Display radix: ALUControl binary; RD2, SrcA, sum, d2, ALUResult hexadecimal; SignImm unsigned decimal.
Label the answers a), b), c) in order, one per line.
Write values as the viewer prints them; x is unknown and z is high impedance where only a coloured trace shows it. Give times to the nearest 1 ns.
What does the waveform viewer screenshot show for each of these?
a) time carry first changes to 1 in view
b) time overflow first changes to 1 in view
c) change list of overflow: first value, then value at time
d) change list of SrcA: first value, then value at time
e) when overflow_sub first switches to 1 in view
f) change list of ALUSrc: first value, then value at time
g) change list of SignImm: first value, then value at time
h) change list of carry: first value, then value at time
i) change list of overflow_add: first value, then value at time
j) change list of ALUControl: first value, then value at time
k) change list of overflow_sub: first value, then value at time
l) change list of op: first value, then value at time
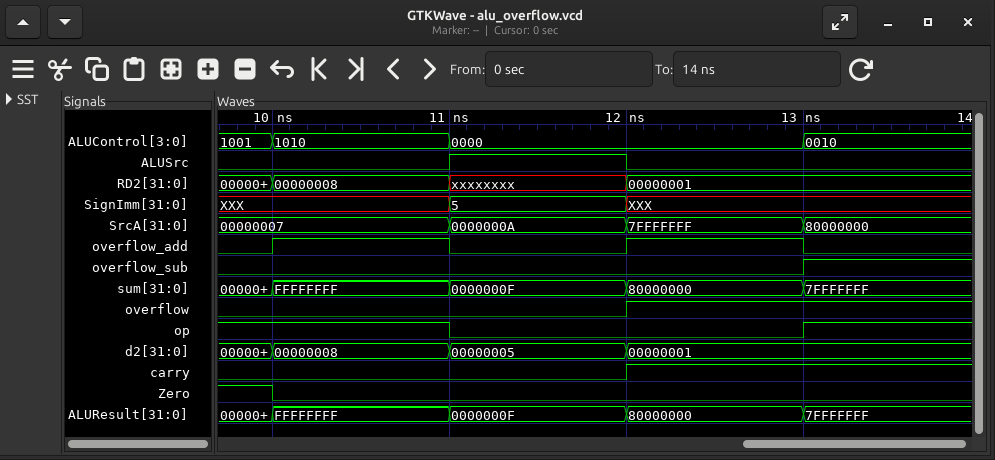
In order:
a) 12 ns
b) 12 ns
c) 0, 1 at 12 ns
d) 00000007, 0000000A at 11 ns, 7FFFFFFF at 12 ns, 80000000 at 13 ns
e) 13 ns
f) 0, 1 at 11 ns, 0 at 12 ns
g) XXX, 5 at 11 ns, XXX at 12 ns
h) 0, 1 at 12 ns
i) 0, 1 at 10 ns, 0 at 11 ns, 1 at 12 ns, 0 at 13 ns
j) 1001, 1010 at 10 ns, 0000 at 11 ns, 0010 at 13 ns
k) 0, 1 at 13 ns
l) 1, 0 at 11 ns, 1 at 13 ns
